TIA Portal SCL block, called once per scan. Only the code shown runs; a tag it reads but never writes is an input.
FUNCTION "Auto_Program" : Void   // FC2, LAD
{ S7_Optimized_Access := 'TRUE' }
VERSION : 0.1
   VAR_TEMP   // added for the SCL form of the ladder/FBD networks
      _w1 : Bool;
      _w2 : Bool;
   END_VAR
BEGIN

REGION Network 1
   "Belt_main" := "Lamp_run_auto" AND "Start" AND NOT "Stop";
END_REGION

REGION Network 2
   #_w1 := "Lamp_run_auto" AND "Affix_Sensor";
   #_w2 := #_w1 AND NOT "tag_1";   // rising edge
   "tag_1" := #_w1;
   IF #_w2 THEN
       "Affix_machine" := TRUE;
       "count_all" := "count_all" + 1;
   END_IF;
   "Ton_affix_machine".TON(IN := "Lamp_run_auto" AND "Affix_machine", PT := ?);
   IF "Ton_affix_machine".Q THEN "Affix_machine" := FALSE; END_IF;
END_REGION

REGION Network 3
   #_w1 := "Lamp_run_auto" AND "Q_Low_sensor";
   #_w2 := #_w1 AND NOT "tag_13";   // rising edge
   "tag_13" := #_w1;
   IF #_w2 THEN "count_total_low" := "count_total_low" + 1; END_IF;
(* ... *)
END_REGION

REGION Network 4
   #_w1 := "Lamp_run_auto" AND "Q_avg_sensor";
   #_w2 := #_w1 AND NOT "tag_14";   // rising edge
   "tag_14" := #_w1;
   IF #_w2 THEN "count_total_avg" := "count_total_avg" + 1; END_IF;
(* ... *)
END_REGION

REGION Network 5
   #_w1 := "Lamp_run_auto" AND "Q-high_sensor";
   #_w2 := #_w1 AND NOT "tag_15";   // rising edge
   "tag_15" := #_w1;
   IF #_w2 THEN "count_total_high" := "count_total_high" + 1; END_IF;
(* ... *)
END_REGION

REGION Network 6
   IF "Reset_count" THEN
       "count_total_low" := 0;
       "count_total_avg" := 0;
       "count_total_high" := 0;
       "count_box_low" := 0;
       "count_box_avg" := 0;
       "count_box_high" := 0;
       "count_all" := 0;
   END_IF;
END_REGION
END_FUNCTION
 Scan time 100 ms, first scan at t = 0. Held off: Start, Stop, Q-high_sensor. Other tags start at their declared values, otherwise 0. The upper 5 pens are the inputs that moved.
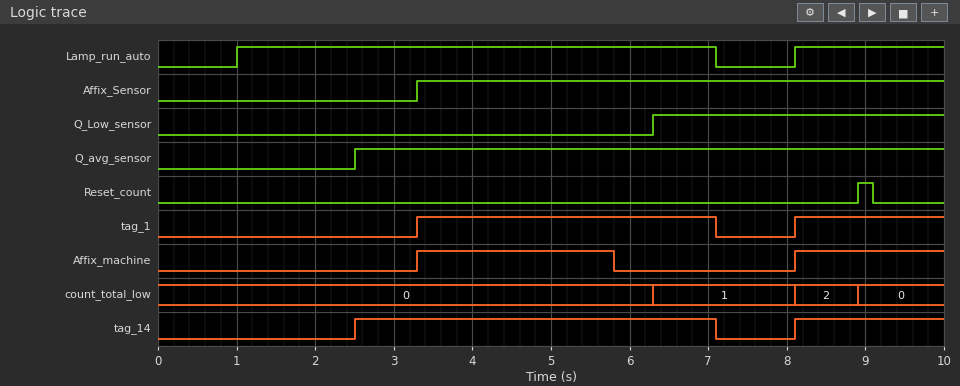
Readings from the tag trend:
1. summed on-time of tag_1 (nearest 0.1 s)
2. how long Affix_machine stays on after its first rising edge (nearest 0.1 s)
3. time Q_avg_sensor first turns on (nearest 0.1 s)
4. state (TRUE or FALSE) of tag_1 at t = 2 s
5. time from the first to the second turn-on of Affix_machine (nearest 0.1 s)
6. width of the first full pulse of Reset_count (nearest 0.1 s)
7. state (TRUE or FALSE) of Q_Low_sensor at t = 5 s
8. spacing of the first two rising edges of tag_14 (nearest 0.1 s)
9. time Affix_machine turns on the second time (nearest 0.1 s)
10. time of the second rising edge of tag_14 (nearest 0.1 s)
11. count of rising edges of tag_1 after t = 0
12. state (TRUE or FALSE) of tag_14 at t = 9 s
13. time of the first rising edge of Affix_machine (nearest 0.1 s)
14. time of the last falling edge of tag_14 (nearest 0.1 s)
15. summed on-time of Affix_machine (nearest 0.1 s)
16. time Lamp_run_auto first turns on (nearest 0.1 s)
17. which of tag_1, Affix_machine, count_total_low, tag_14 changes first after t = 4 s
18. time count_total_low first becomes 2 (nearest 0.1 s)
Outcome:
5.7 s
2.5 s
2.5 s
FALSE
4.8 s
0.2 s
FALSE
5.6 s
8.1 s
8.1 s
2
TRUE
3.3 s
7.1 s
4.4 s
1.0 s
Affix_machine
8.1 s
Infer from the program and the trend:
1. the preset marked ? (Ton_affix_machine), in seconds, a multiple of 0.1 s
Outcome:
2.5 s
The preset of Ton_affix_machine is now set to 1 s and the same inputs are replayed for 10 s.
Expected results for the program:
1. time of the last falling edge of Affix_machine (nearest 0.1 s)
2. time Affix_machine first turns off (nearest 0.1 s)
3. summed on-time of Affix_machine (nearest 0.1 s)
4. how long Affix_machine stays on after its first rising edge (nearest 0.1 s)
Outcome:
9.1 s
4.3 s
2.0 s
1.0 s
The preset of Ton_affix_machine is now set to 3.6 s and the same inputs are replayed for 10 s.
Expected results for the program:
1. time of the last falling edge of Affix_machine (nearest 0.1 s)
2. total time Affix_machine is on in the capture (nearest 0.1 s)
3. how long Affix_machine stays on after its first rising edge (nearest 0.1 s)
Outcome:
6.9 s
5.5 s
3.6 s
